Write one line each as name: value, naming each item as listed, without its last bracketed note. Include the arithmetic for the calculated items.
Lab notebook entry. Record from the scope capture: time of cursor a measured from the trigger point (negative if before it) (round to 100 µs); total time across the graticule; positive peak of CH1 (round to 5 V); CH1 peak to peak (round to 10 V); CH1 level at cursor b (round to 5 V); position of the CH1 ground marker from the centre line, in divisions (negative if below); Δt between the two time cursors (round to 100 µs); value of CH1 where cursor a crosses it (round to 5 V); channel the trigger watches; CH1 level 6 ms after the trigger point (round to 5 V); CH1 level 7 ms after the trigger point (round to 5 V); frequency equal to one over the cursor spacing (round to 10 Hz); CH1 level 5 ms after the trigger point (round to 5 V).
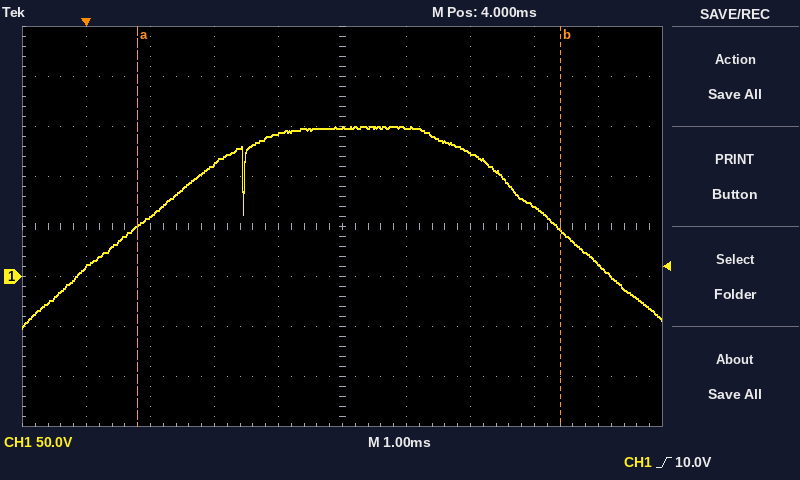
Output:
time of cursor a measured from the trigger point (negative if before it): +800 µs
total time across the graticule: 10 ms
positive peak of CH1: 150 V
CH1 peak to peak: 200 V
CH1 level at cursor b: 45 V
position of the CH1 ground marker from the centre line, in divisions: -1.0 div
Δt between the two time cursors: 6.6 ms
value of CH1 where cursor a crosses it: 50 V
channel the trigger watches: CH1
CH1 level 6 ms after the trigger point: 125 V
CH1 level 7 ms after the trigger point: 70 V
frequency equal to one over the cursor spacing: 1 / 6.6 ms ≈ 150 Hz
CH1 level 5 ms after the trigger point: 150 V
